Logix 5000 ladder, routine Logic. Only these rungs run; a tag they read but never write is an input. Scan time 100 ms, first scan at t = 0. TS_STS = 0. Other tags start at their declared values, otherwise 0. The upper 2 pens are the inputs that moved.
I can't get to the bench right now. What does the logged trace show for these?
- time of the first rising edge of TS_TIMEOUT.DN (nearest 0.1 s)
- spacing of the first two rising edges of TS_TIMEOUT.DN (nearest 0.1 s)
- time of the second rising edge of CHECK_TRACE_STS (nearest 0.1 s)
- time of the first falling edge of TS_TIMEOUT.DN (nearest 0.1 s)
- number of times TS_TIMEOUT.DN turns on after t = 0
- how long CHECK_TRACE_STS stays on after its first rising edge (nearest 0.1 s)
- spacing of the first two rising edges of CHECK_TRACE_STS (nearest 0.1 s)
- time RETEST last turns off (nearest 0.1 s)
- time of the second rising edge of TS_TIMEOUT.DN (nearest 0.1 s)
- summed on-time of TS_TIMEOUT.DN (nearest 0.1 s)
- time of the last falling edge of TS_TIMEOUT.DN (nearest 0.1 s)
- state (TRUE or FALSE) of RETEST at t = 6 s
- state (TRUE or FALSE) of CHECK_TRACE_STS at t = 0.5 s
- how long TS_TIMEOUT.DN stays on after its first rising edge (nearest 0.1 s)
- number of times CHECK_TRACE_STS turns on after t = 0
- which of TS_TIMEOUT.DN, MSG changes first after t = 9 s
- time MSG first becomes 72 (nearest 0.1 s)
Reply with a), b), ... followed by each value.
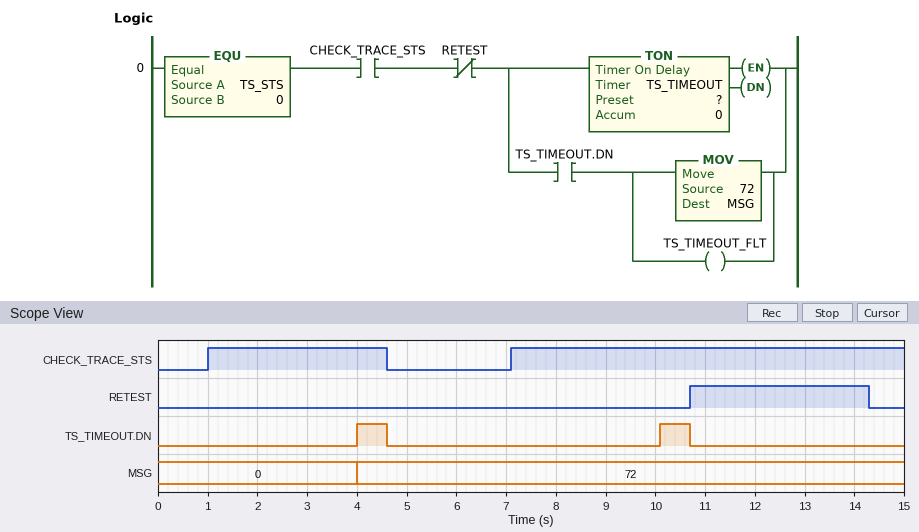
a) 4.0 s
b) 6.1 s
c) 7.1 s
d) 4.6 s
e) 2
f) 3.6 s
g) 6.1 s
h) 14.3 s
i) 10.1 s
j) 1.2 s
k) 10.7 s
l) FALSE
m) FALSE
n) 0.6 s
o) 2
p) TS_TIMEOUT.DN
q) 4.0 s
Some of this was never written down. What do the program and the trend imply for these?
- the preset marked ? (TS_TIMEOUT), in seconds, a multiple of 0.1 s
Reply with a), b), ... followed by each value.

a) 3.0 s
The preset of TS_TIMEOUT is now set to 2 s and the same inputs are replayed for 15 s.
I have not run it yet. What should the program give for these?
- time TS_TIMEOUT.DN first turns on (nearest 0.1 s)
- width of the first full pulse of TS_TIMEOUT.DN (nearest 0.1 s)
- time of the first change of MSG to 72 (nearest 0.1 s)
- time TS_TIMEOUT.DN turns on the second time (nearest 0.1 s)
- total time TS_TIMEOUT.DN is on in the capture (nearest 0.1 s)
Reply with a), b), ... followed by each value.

a) 3.0 s
b) 1.6 s
c) 3.0 s
d) 9.1 s
e) 3.2 s
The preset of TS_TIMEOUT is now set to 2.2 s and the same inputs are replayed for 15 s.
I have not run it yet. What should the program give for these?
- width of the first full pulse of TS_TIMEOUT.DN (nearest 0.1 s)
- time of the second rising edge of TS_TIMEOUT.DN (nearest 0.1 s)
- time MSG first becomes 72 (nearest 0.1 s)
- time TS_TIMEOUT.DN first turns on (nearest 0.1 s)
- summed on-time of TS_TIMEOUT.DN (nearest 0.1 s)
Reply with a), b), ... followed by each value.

a) 1.4 s
b) 9.3 s
c) 3.2 s
d) 3.2 s
e) 2.8 s
